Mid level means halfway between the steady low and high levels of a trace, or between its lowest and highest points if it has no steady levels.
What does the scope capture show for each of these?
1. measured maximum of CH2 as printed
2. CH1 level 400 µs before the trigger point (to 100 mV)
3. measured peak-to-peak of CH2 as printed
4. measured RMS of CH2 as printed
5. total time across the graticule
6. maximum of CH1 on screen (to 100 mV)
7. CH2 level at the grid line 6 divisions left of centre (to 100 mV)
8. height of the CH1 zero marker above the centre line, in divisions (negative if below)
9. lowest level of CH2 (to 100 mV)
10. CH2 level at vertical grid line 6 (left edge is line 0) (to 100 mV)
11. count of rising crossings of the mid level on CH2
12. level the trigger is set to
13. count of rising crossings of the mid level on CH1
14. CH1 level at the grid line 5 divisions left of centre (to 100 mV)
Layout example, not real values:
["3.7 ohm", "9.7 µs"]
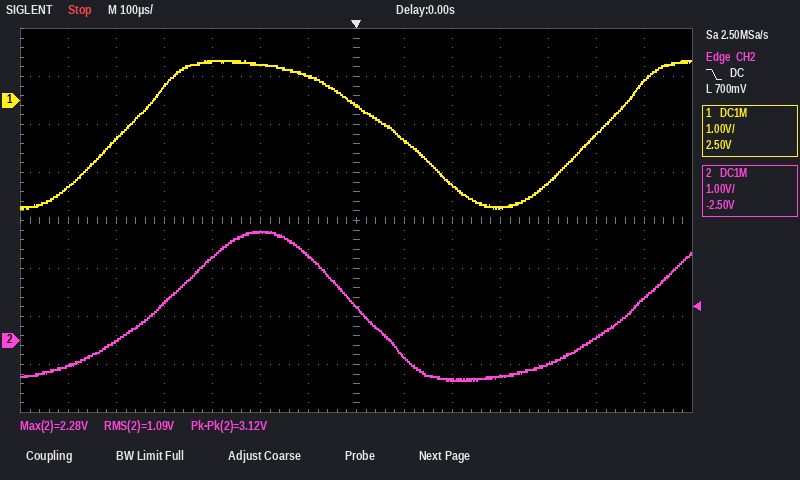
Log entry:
["2.28 V", "300 mV", "3.12 V", "1.09 V", "1.4 ms", "800 mV", "-500 mV", "+2.5 div", "-800 mV", "1.8 V", "2", "700 mV", "2", "-800 mV"]
